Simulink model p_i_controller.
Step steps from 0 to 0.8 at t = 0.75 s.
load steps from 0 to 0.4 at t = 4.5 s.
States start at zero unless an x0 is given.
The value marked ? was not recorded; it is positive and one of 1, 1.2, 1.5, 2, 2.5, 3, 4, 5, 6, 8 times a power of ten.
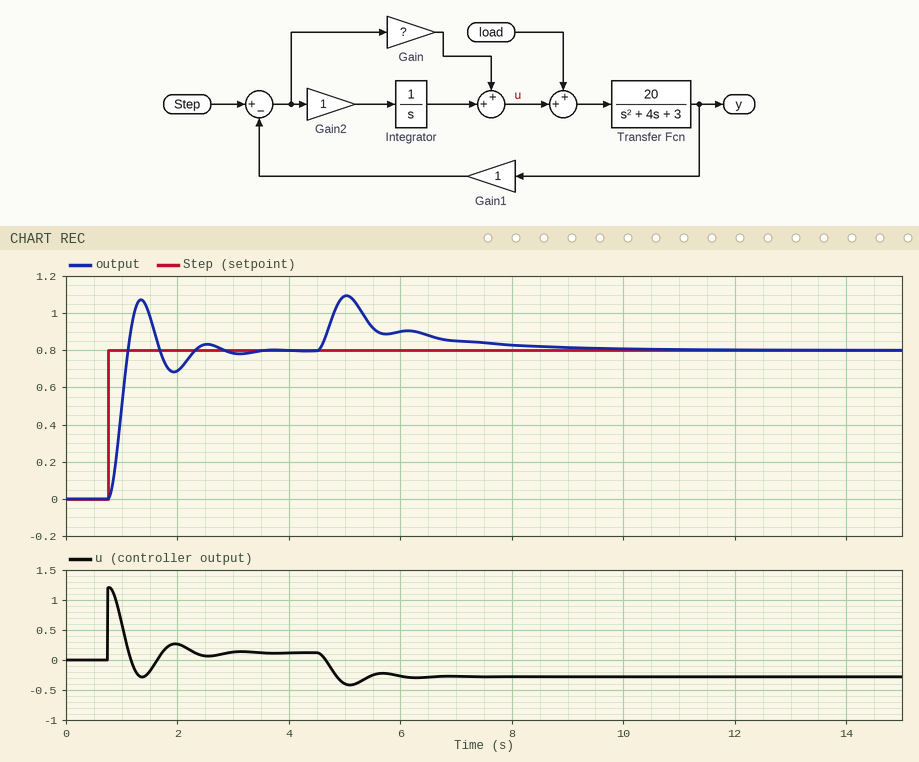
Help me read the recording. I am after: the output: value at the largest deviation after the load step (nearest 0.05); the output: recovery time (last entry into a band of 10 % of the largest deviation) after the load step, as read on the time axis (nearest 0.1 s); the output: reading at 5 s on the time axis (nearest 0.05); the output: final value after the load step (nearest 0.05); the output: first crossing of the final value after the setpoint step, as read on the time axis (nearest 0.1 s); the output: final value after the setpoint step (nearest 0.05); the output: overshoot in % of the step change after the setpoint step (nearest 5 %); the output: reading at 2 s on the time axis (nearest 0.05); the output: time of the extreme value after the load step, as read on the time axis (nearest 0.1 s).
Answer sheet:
1.10
7.9 s
1.10
0.80
1.1 s
0.80
35 %
0.70
5.0 s
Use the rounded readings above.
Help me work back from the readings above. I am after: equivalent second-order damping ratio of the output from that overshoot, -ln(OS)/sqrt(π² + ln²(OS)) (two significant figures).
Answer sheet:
0.32
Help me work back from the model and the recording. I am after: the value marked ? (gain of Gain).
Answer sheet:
1.5
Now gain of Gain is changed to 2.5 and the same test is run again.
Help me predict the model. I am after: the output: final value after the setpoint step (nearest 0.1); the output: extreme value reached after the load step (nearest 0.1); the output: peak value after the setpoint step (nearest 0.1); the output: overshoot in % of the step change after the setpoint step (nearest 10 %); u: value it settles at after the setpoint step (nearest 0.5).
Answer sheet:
0.8
1.0
1.1
40 %
0.0
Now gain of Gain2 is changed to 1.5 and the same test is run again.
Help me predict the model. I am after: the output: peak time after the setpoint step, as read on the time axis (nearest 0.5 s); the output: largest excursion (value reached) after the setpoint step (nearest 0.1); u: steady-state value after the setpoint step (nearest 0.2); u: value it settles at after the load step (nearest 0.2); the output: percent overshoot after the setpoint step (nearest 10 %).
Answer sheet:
1.5 s
1.1
0.2
-0.2
40 %
